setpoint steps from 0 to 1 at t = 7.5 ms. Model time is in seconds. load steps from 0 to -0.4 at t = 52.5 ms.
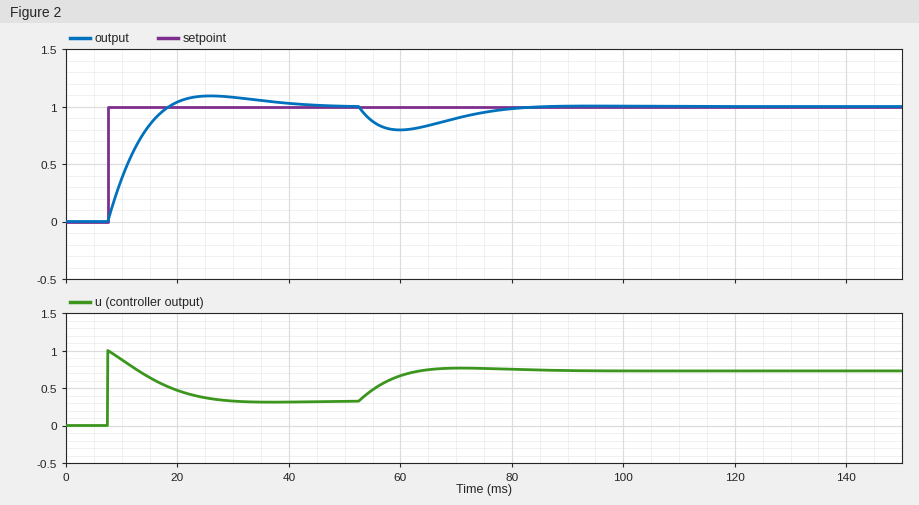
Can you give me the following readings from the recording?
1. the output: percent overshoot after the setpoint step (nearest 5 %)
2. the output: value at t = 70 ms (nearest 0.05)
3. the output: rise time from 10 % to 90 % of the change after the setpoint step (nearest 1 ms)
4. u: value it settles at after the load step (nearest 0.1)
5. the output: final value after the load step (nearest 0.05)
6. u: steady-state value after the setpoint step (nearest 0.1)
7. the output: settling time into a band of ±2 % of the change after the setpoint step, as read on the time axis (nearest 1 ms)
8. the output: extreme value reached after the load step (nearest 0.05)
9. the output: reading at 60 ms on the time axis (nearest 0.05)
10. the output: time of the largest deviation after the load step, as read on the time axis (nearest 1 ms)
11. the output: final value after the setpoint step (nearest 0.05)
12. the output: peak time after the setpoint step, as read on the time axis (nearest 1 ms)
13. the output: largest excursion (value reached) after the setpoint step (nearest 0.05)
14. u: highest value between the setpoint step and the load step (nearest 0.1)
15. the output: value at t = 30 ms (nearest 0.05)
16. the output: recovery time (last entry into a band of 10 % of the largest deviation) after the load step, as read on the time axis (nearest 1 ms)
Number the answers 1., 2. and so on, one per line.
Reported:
1. 10 %
2. 0.90
3. 8 ms
4. 0.7
5. 1.00
6. 0.3
7. 42 ms
8. 0.80
9. 0.80
10. 60 ms
11. 1.00
12. 26 ms
13. 1.10
14. 1.0
15. 1.10
16. 80 ms
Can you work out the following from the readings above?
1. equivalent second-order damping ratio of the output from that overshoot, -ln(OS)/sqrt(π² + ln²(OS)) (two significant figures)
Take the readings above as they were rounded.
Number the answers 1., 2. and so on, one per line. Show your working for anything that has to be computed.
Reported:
1. ln(0.1) = -2.303; 2.303 / sqrt(9.870 + 5.302) = 0.59
